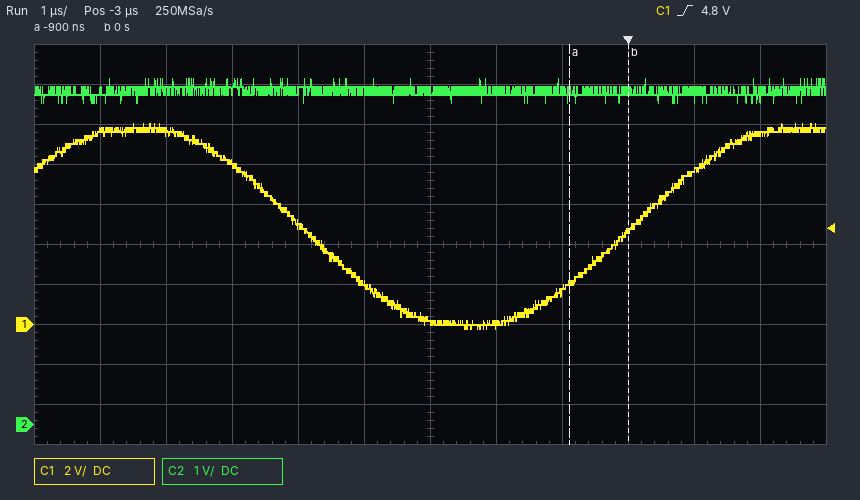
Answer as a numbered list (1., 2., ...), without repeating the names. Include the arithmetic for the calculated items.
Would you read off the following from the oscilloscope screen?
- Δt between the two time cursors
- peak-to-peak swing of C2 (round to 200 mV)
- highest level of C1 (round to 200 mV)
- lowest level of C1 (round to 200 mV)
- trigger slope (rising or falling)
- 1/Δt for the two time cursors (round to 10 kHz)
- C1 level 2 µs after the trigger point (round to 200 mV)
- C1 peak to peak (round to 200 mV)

1. 0 s − (-900 ns) = 900 ns
2. 600 mV
3. 10.0 V
4. -200 mV
5. rising
6. 1 / 900 ns ≈ 1.11 MHz
7. 9.6 V
8. 10.0 V − (-200 mV) = 10.2 V
